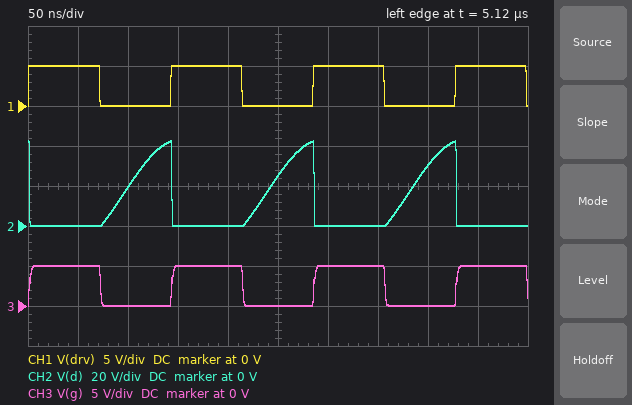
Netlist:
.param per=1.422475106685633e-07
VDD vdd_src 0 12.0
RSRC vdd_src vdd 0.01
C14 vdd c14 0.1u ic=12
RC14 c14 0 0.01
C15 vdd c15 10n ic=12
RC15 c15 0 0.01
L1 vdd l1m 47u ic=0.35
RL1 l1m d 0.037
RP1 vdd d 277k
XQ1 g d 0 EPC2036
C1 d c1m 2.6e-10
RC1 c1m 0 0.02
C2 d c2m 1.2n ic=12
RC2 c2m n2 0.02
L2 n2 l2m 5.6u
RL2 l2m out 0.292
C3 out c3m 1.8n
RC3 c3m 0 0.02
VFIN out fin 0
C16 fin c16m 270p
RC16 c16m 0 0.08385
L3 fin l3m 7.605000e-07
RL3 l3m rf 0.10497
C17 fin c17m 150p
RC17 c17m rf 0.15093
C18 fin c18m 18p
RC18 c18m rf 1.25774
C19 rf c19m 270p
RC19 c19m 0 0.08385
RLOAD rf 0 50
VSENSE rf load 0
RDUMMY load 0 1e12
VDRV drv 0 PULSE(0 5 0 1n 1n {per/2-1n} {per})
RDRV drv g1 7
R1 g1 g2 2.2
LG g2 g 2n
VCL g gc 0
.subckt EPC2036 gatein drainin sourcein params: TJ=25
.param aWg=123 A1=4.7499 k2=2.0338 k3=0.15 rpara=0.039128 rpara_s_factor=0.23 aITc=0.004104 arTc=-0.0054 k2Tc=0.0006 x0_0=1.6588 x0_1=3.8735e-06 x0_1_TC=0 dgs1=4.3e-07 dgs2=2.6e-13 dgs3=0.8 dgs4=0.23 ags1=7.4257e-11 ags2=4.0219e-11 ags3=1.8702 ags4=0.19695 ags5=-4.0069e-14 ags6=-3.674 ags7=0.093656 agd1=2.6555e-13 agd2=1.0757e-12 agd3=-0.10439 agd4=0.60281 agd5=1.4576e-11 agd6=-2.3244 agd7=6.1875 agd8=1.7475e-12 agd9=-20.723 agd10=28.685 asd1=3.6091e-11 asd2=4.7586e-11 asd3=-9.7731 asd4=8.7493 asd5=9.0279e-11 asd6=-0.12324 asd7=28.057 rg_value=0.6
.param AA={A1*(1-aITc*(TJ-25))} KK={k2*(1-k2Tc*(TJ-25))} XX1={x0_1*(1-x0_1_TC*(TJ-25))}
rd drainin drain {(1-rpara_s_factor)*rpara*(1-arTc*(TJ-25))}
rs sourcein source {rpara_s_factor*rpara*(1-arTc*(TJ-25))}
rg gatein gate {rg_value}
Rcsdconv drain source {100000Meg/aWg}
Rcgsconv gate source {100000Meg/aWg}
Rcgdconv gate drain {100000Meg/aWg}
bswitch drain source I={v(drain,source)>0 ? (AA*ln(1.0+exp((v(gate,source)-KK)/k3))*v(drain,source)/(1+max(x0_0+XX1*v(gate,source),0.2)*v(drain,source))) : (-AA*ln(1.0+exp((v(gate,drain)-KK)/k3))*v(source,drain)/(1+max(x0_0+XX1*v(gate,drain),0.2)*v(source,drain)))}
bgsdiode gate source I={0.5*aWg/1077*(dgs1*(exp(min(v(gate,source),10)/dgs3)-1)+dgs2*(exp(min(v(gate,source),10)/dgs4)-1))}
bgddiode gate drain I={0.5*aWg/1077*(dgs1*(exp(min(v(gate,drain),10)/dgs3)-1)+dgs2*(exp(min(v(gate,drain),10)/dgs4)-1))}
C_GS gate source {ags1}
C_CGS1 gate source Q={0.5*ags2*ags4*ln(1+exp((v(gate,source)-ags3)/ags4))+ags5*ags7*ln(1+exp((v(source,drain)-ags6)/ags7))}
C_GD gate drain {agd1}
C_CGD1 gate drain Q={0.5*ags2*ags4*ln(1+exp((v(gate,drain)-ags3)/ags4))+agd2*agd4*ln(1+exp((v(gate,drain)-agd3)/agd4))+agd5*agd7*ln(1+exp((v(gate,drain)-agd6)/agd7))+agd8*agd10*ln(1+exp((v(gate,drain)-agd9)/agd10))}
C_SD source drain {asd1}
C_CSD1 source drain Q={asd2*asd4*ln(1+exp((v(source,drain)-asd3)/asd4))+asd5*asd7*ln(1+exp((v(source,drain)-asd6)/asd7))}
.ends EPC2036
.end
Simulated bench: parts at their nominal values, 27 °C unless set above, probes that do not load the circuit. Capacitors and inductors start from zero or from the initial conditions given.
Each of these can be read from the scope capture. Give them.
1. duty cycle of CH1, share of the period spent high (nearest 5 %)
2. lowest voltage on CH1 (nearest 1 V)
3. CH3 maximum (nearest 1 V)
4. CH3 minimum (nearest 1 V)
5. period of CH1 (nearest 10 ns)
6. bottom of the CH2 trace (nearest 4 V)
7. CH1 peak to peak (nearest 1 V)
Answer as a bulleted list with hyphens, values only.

- 50 %
- 0 V
- 5 V
- 0 V
- 140 ns
- 0 V
- 5 V
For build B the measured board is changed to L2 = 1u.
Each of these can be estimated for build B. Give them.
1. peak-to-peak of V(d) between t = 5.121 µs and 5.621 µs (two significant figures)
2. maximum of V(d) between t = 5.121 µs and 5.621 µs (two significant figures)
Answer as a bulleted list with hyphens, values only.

- 66 V
- 64 V
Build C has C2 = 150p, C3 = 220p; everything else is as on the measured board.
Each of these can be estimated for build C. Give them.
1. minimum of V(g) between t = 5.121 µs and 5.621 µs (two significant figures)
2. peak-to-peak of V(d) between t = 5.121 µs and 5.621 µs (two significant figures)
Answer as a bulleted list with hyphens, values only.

- -2.4 mV
- 33 V
